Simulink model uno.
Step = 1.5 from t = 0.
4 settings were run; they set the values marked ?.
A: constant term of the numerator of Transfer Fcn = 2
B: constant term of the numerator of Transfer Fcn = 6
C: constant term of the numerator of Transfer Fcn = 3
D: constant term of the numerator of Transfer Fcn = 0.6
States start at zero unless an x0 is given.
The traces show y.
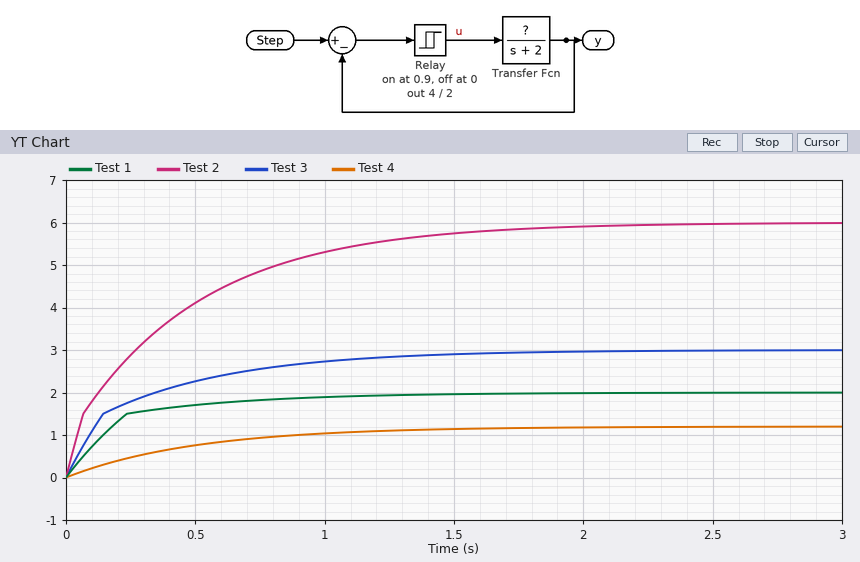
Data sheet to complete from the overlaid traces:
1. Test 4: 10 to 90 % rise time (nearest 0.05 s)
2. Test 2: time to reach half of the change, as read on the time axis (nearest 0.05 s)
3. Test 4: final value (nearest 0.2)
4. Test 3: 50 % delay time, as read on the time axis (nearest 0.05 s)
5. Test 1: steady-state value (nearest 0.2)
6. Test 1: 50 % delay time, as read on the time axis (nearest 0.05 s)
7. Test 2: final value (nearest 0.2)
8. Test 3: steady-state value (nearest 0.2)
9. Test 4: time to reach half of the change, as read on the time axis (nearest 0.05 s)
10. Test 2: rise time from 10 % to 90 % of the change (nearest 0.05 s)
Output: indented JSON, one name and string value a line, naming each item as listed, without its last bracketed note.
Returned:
{
  "Test 4: 10 to 90 % rise time": "1.10 s",
  "Test 2: time to reach half of the change, as read on the time axis": "0.25 s",
  "Test 4: final value": "1.2",
  "Test 3: 50 % delay time, as read on the time axis": "0.15 s",
  "Test 1: steady-state value": "2.0",
  "Test 1: 50 % delay time, as read on the time axis": "0.15 s",
  "Test 2: final value": "6.0",
  "Test 3: steady-state value": "3.0",
  "Test 4: time to reach half of the change, as read on the time axis": "0.35 s",
  "Test 2: rise time from 10 % to 90 % of the change": "1.05 s"
}
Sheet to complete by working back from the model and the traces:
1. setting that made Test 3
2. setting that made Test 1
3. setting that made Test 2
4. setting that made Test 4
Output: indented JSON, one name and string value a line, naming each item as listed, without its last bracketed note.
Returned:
{
  "setting that made Test 3": "C",
  "setting that made Test 1": "A",
  "setting that made Test 2": "B",
  "setting that made Test 4": "D"
}
